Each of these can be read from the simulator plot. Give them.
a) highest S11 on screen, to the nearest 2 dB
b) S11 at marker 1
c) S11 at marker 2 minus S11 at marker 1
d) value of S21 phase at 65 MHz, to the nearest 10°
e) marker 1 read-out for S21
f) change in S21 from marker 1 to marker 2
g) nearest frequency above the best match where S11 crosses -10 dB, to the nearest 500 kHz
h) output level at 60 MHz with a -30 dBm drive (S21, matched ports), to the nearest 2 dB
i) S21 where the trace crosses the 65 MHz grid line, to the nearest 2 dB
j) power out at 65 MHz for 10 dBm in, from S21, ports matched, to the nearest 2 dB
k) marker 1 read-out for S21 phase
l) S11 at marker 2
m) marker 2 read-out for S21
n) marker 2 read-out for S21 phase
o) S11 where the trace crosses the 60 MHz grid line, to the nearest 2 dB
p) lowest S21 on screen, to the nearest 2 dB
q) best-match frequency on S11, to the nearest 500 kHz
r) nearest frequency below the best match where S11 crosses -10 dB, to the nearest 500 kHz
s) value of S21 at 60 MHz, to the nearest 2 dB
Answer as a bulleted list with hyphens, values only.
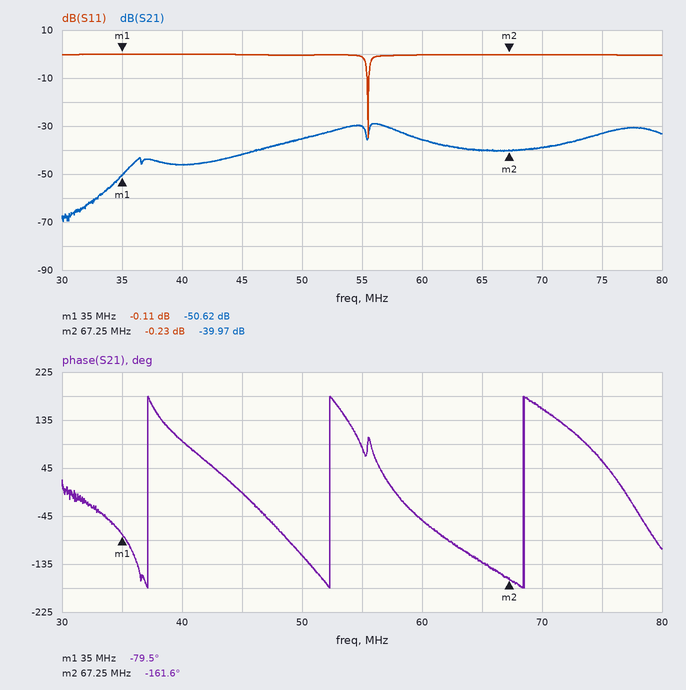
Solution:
- 0 dB
- -0.11 dB
- -0.12 dB
- -130°
- -50.62 dB
- 10.65 dB
- 55.5 MHz
- -66 dBm
- -40 dB
- -30 dBm
- -79.5°
- -0.23 dB
- -39.97 dB
- -161.6°
- 0 dB
- -70 dB
- 55.5 MHz
- 55.5 MHz
- -36 dB
